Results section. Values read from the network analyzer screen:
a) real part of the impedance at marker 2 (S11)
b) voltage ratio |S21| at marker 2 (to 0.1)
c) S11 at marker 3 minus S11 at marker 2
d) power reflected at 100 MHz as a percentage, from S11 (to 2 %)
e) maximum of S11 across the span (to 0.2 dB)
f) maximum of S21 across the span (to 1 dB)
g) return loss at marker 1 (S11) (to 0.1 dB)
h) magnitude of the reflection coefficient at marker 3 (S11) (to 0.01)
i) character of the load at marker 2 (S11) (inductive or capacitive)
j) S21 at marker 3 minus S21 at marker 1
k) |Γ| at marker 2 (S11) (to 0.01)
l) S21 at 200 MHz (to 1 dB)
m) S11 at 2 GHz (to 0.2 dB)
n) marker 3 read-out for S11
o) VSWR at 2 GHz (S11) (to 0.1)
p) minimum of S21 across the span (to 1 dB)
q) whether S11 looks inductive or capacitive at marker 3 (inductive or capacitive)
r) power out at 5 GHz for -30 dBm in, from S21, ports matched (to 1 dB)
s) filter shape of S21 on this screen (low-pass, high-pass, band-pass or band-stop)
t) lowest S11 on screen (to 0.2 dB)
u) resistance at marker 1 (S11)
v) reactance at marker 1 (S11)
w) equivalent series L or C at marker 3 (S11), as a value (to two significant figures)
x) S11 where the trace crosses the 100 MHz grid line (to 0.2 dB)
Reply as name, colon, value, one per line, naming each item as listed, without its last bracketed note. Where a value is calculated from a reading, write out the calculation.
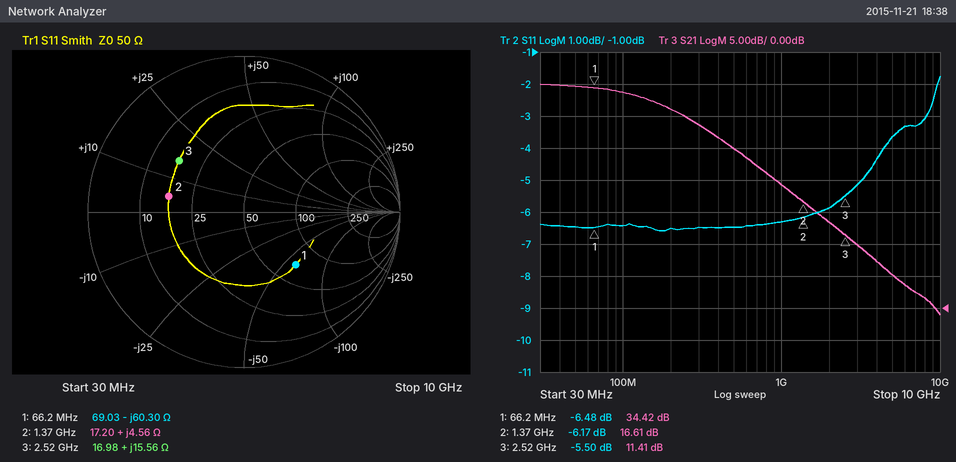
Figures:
real part of the impedance at marker 2: 17.20 Ω
voltage ratio |S21| at marker 2: 10^(16.61/20) ≈ 6.8
S11 at marker 3 minus S11 at marker 2: -5.5 − (-6.17) = 0.67 dB
power reflected at 100 MHz as a percentage, from S11: 10^(-6.4/10) ≈ 22.9 %, so 22 % to the nearest 2 %
maximum of S11 across the span: -1.8 dB
maximum of S21 across the span: 35 dB
return loss at marker 1 (S11): 6.5 dB
magnitude of the reflection coefficient at marker 3 (S11): 10^(-5.5/20) ≈ 0.53
character of the load at marker 2 (S11): inductive
S21 at marker 3 minus S21 at marker 1: 11.41 − (34.42) = -23.01 dB
|Γ| at marker 2 (S11): 0.49
S21 at 200 MHz: 31 dB
S11 at 2 GHz: -5.8 dB
marker 3 read-out for S11: -5.50 dB
VSWR at 2 GHz (S11): |Γ| = 10^(-5.8/20) = 0.5129; VSWR = (1 + 0.5129)/(1 − 0.5129) ≈ 3.1
minimum of S21 across the span: -1 dB
whether S11 looks inductive or capacitive at marker 3: inductive
power out at 5 GHz for -30 dBm in, from S21, ports matched: -30 dBm + (5 dB) = -25 dBm
filter shape of S21 on this screen: low-pass
lowest S11 on screen: -6.6 dB
resistance at marker 1: 69.03 Ω
reactance at marker 1: -60.30 Ω
equivalent series L or C at marker 3 (S11), as a value: L = 15.56 Ω/(2π × 2.52 GHz) ≈ 983 pH, so 980 pH to two significant figures
S11 where the trace crosses the 100 MHz grid line: -6.4 dB
